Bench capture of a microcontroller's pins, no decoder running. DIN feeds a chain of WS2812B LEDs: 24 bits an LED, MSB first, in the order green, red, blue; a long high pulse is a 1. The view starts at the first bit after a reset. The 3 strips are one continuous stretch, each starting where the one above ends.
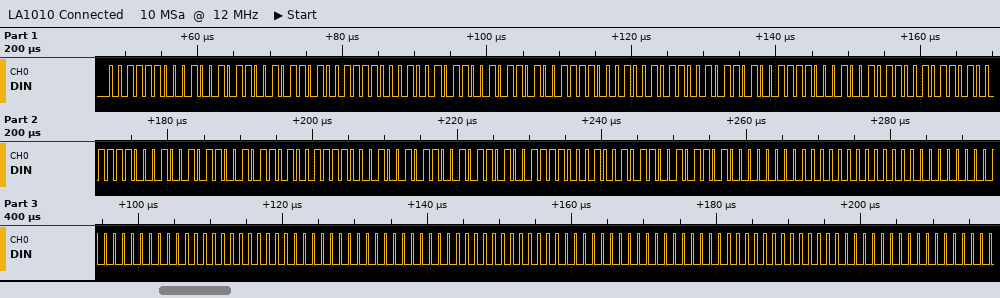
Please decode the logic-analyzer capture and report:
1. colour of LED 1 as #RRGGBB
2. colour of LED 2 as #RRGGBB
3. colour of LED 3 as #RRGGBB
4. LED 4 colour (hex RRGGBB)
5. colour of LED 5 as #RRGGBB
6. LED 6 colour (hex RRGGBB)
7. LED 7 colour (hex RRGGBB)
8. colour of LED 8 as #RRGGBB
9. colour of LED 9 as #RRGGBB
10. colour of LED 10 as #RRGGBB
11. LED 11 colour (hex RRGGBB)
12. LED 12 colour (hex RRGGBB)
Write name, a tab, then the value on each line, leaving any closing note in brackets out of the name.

colour of LED 1 as #RRGGBB	#4B3C2D
colour of LED 2 as #RRGGBB	#4B3C2D
colour of LED 3 as #RRGGBB	#4B3C2D
LED 4 colour	#4B3C2D
colour of LED 5 as #RRGGBB	#4B3C2D
LED 6 colour	#4B3C2D
LED 7 colour	#4B3C2D
colour of LED 8 as #RRGGBB	#000000
colour of LED 9 as #RRGGBB	#000000
colour of LED 10 as #RRGGBB	#000000
LED 11 colour	#000000
LED 12 colour	#000000
